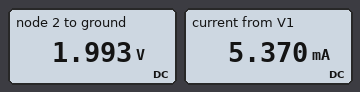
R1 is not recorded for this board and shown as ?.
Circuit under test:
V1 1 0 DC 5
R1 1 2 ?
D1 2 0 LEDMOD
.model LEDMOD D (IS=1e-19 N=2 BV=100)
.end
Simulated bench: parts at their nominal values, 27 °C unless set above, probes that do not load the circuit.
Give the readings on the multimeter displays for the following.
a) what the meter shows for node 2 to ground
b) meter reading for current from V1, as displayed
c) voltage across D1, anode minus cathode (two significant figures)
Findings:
1.993 V
5.370 mA
2.0 V
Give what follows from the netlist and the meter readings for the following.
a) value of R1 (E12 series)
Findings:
560 Ω
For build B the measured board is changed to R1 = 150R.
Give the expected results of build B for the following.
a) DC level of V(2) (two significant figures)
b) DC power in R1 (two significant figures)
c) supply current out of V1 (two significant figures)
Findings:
2.1 V
58 mW
20 mA
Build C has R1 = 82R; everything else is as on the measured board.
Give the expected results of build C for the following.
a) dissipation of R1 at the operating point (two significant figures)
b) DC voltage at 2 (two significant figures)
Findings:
100 mW
2.1 V
